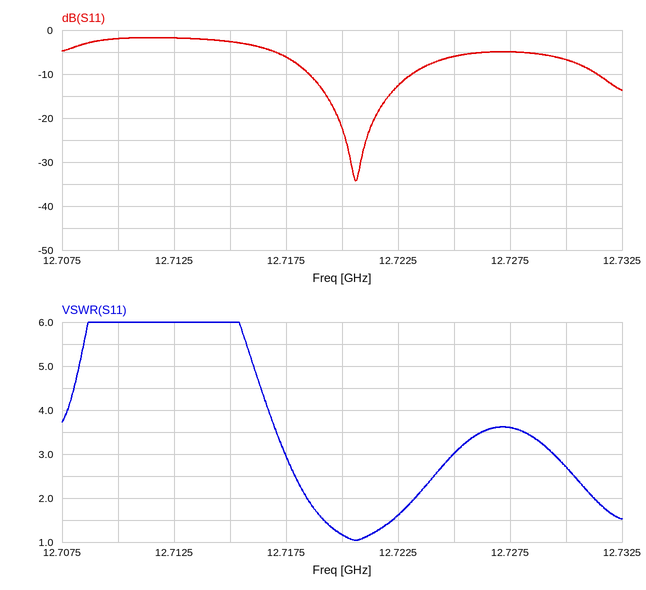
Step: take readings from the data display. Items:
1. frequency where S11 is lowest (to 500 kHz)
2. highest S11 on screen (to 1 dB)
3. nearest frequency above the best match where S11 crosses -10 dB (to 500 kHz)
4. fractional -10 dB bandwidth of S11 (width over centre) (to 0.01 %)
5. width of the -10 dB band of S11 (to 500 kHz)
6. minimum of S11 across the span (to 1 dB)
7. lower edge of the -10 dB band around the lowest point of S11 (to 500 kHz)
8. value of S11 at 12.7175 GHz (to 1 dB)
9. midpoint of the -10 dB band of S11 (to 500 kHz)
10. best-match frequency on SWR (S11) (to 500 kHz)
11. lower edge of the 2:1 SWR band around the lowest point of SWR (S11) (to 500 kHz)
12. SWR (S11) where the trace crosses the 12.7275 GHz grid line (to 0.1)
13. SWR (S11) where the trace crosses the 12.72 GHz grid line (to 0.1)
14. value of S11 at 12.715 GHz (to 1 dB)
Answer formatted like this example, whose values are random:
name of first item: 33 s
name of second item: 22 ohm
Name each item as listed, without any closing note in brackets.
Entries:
frequency where S11 is lowest: 12.7205 GHz
highest S11 on screen: -2 dB
nearest frequency above the best match where S11 crosses -10 dB: 12.7230 GHz
fractional -10 dB bandwidth of S11 (width over centre): 0.04 %
width of the -10 dB band of S11: 4.5 MHz
minimum of S11 across the span: -34 dB
lower edge of the -10 dB band around the lowest point of S11: 12.7185 GHz
value of S11 at 12.7175 GHz: -6 dB
midpoint of the -10 dB band of S11: 12.7210 GHz
best-match frequency on SWR (S11): 12.7205 GHz
lower edge of the 2:1 SWR band around the lowest point of SWR (S11): 12.7185 GHz
SWR (S11) where the trace crosses the 12.7275 GHz grid line: 3.6
SWR (S11) where the trace crosses the 12.72 GHz grid line: 1.2
value of S11 at 12.715 GHz: -3 dB
